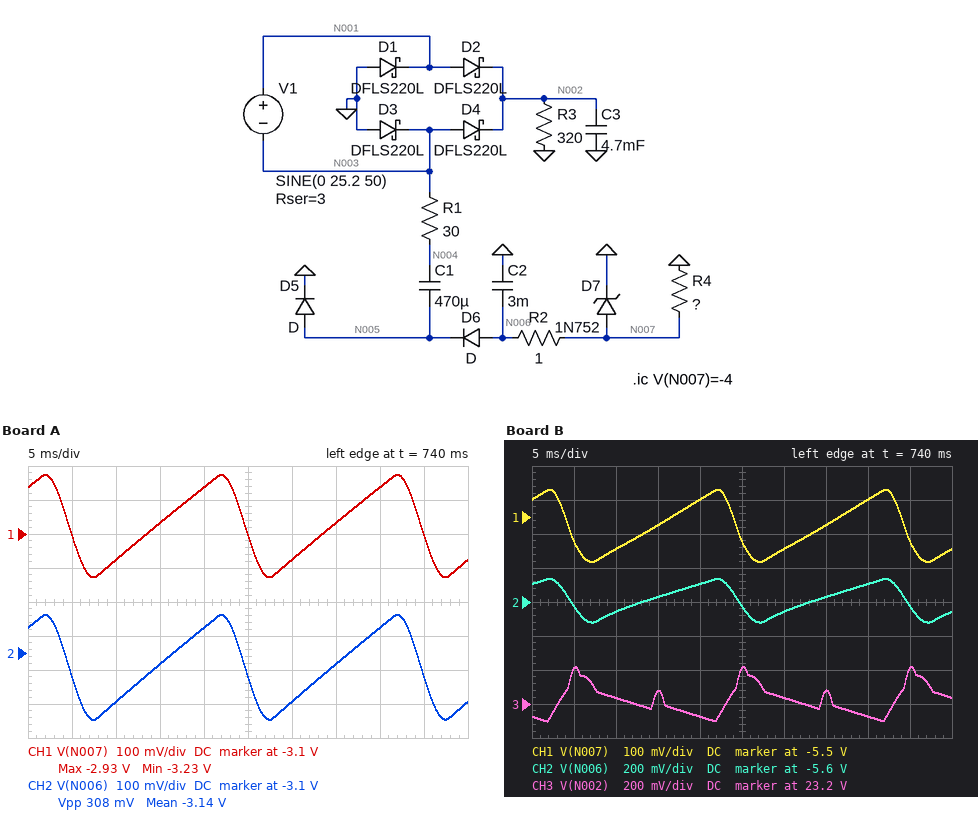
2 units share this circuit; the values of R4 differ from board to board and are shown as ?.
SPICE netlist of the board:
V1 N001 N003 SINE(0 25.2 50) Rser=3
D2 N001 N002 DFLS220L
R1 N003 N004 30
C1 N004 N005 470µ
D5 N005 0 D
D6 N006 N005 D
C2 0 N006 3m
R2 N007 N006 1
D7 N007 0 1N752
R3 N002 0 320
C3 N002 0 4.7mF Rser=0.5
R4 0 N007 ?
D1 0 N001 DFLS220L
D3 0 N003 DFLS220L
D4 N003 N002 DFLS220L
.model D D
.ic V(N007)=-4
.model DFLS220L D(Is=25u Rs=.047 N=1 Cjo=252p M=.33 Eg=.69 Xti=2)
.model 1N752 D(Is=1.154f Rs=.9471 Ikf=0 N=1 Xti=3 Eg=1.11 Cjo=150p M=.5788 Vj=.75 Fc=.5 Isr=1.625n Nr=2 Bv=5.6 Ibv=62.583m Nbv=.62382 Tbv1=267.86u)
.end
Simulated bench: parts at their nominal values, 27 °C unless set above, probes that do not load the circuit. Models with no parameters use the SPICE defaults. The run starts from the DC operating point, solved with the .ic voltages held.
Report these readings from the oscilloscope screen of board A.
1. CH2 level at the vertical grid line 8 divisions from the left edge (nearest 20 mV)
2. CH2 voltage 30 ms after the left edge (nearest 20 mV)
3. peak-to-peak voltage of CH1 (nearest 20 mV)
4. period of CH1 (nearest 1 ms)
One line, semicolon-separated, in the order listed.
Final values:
-3.02 V; -3.24 V; 300 mV; 20 ms
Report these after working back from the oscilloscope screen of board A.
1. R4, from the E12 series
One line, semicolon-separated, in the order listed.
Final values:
47 Ω
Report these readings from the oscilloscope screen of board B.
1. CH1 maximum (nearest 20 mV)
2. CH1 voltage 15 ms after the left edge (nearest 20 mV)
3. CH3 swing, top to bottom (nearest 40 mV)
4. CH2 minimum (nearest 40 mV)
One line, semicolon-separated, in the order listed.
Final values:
-5.42 V; -5.52 V; 320 mV; -5.72 V
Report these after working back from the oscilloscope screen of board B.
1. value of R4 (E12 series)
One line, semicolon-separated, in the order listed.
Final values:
120 Ω
